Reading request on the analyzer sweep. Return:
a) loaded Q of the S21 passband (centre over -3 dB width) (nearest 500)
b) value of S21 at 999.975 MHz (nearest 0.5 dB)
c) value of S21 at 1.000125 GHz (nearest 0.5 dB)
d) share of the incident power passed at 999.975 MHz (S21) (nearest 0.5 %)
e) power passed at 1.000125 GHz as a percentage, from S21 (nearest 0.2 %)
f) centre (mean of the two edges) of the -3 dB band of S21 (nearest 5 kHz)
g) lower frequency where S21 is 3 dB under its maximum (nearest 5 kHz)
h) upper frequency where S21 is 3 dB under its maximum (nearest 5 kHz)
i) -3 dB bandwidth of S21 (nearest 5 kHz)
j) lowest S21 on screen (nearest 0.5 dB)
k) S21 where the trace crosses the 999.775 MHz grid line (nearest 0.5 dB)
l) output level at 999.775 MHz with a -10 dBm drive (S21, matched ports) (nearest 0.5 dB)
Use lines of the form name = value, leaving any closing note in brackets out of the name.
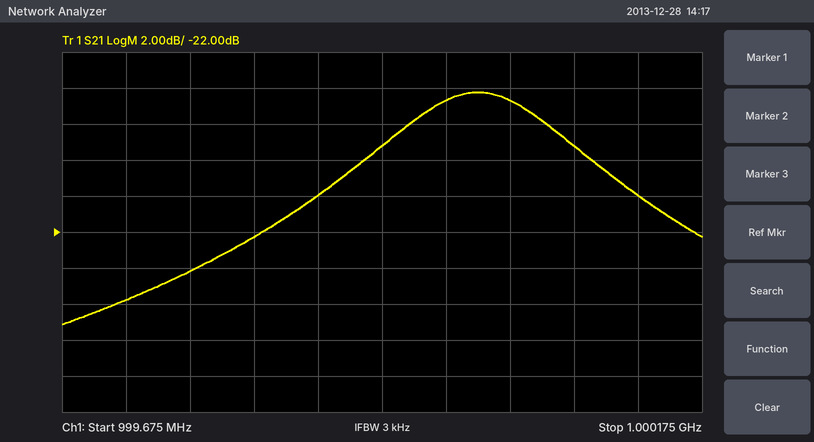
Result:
loaded Q of the S21 passband (centre over -3 dB width) = 6500
value of S21 at 999.975 MHz = -14.5 dB
value of S21 at 1.000125 GHz = -20.0 dB
share of the incident power passed at 999.975 MHz (S21) = 3.5 %
power passed at 1.000125 GHz as a percentage, from S21 = 1.0 %
centre (mean of the two edges) of the -3 dB band of S21 = 1.000000 GHz
lower frequency where S21 is 3 dB under its maximum = 999.925 MHz
upper frequency where S21 is 3 dB under its maximum = 1.000075 GHz
-3 dB bandwidth of S21 = 150 kHz
lowest S21 on screen = -27.0 dB
S21 where the trace crosses the 999.775 MHz grid line = -24.0 dB
output level at 999.775 MHz with a -10 dBm drive (S21, matched ports) = -34.0 dBm
